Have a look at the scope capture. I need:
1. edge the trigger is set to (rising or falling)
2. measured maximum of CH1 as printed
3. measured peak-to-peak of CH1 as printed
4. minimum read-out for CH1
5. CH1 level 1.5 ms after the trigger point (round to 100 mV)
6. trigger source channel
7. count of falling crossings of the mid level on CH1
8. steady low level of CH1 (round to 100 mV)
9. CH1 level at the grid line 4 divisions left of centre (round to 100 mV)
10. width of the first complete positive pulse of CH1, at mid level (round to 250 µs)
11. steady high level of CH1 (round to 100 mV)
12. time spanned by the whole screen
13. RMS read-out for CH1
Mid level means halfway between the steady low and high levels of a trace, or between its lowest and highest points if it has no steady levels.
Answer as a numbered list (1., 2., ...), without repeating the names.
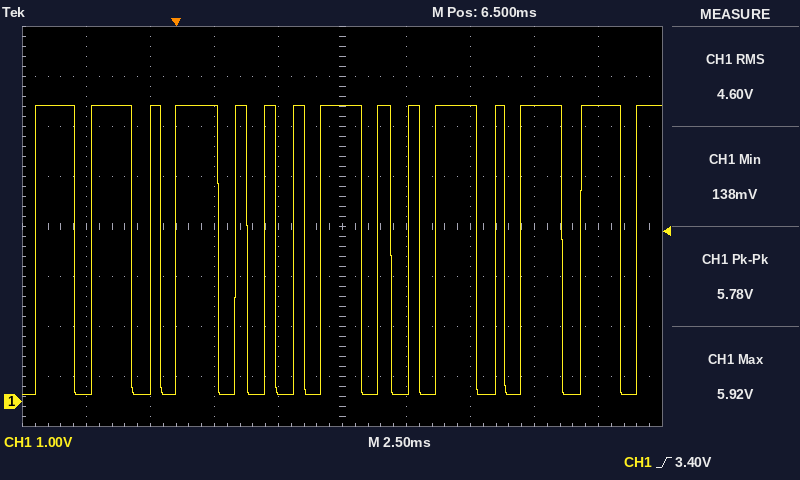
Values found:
1. rising
2. 5.92 V
3. 5.78 V
4. 138 mV
5. 5.9 V
6. CH1
7. 14
8. 100 mV
9. 100 mV
10. 1.50 ms
11. 5.9 V
12. 25 ms
13. 4.60 V
